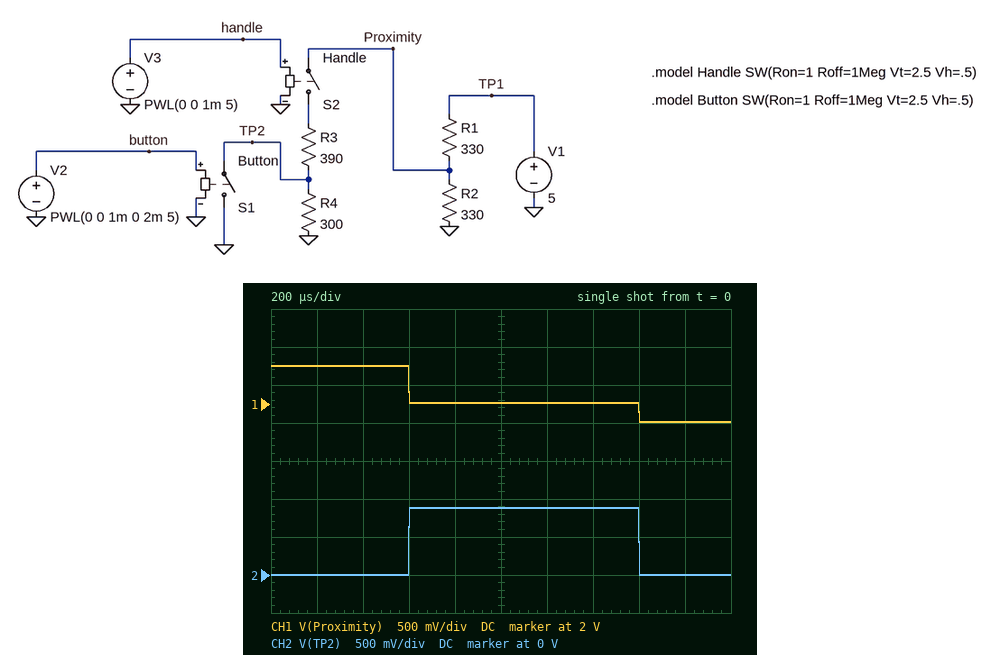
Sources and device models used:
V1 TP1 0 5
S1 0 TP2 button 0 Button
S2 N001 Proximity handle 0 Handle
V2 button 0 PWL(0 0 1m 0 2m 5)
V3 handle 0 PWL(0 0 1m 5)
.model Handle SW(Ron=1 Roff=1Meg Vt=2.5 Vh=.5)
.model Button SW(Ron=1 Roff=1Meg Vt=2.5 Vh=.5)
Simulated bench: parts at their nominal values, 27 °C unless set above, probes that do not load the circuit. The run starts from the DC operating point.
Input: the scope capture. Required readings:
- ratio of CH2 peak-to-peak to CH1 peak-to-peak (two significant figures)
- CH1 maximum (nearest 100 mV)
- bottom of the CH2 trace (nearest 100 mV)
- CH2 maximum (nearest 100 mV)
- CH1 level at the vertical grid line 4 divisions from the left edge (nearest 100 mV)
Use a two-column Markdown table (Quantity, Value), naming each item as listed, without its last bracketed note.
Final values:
| Quantity | Value |
|---|---|
| ratio of CH2 peak-to-peak to CH1 peak-to-peak | 1.2 |
| CH1 maximum | 2.5 V |
| bottom of the CH2 trace | 0 V |
| CH2 maximum | 900 mV |
| CH1 level at the vertical grid line 4 divisions from the left edge | 2.0 V |
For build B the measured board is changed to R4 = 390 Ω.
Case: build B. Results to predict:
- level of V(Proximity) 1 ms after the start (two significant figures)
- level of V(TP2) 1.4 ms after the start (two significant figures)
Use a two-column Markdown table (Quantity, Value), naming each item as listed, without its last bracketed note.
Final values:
| Quantity | Value |
|---|---|
| level of V(Proximity) 1 ms after the start | 2.1 V |
| level of V(TP2) 1.4 ms after the start | 1.0 V |
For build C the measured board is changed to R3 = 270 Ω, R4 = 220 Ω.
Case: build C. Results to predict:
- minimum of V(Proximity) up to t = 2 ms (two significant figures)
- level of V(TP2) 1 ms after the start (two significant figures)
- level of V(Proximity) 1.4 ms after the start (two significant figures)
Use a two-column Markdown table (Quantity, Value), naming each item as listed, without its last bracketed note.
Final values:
| Quantity | Value |
|---|---|
| minimum of V(Proximity) up to t = 2 ms | 1.6 V |
| level of V(TP2) 1 ms after the start | 840 mV |
| level of V(Proximity) 1.4 ms after the start | 1.9 V |
